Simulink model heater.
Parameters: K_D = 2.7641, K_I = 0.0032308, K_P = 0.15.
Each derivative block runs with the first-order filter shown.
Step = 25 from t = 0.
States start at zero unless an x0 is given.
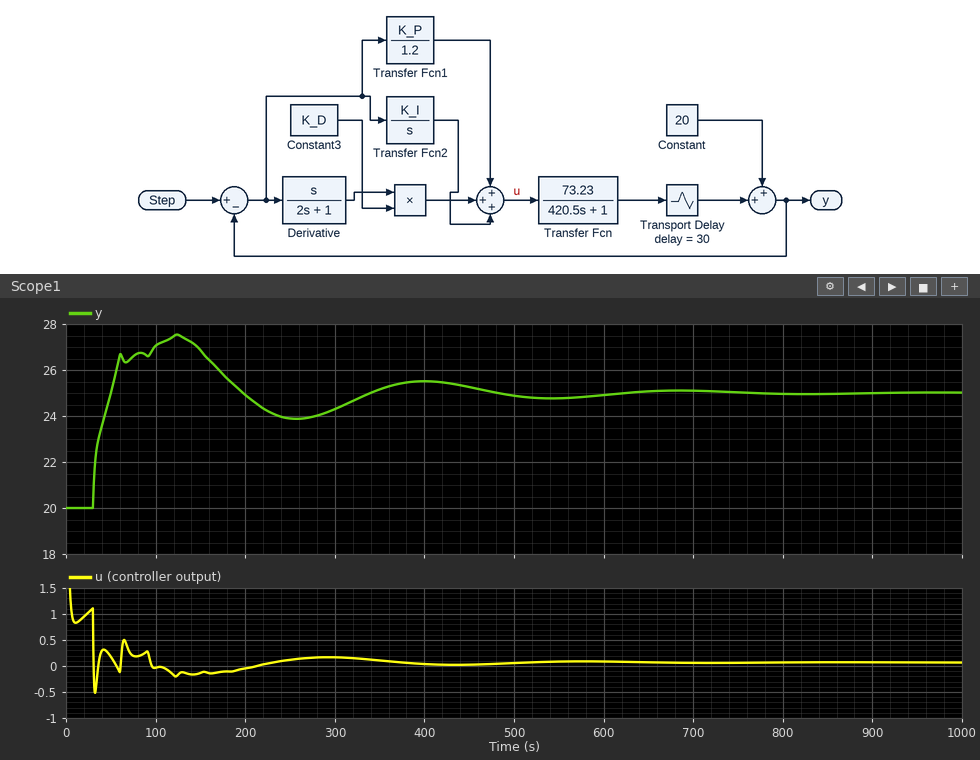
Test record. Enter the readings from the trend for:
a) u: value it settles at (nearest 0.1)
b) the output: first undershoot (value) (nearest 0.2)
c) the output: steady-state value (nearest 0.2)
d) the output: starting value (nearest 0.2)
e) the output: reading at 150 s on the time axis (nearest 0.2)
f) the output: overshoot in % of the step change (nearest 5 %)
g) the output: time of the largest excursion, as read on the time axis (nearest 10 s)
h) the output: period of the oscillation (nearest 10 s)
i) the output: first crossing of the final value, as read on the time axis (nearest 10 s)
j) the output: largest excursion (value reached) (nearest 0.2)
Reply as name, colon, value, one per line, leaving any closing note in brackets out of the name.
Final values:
u: value it settles at: 0.1
the output: first undershoot (value): 23.8
the output: steady-state value: 25.0
the output: starting value: 20.0
the output: reading at 150 s on the time axis: 26.8
the output: overshoot in % of the step change: 50 %
the output: time of the largest excursion, as read on the time axis: 120 s
the output: period of the oscillation: 280 s
the output: first crossing of the final value, as read on the time axis: 50 s
the output: largest excursion (value reached): 27.6
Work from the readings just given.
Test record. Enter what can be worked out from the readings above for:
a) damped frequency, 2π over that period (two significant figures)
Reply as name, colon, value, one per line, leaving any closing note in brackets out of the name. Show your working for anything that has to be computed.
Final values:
damped frequency, 2π over that period: 2π / 280 = 0.022 rad/s
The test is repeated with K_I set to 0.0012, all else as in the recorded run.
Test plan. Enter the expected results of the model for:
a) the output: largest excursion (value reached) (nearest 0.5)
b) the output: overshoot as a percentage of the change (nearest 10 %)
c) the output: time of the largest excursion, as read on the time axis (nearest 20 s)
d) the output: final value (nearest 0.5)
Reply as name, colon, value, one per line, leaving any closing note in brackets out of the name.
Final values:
the output: largest excursion (value reached): 26.0
the output: overshoot as a percentage of the change: 20 %
the output: time of the largest excursion, as read on the time axis: 140 s
the output: final value: 25.0
